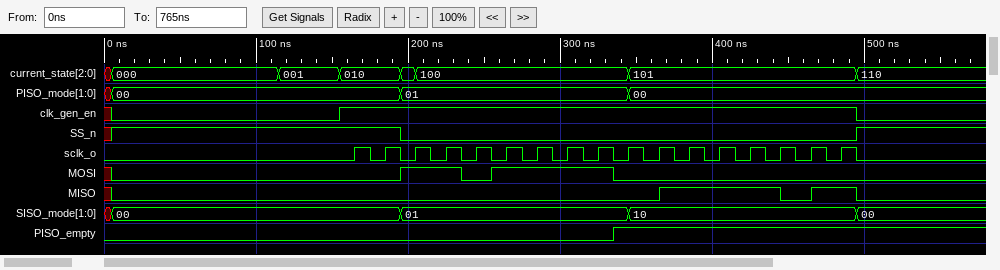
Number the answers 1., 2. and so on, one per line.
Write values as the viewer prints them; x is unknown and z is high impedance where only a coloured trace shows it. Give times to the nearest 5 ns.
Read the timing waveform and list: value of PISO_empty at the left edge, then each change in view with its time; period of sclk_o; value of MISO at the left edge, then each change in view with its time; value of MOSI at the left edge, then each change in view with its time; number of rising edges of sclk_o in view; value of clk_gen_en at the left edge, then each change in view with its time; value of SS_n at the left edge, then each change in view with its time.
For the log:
1. 0, 1 at 335 ns
2. 20 ns
3. x, 0 at 5 ns, 1 at 365 ns, 0 at 445 ns, 1 at 465 ns, 0 at 495 ns
4. x, 0 at 5 ns, 1 at 195 ns, 0 at 235 ns, 1 at 255 ns, 0 at 335 ns
5. 17
6. x, 0 at 5 ns, 1 at 155 ns, 0 at 495 ns
7. x, 1 at 5 ns, 0 at 195 ns, 1 at 495 ns
